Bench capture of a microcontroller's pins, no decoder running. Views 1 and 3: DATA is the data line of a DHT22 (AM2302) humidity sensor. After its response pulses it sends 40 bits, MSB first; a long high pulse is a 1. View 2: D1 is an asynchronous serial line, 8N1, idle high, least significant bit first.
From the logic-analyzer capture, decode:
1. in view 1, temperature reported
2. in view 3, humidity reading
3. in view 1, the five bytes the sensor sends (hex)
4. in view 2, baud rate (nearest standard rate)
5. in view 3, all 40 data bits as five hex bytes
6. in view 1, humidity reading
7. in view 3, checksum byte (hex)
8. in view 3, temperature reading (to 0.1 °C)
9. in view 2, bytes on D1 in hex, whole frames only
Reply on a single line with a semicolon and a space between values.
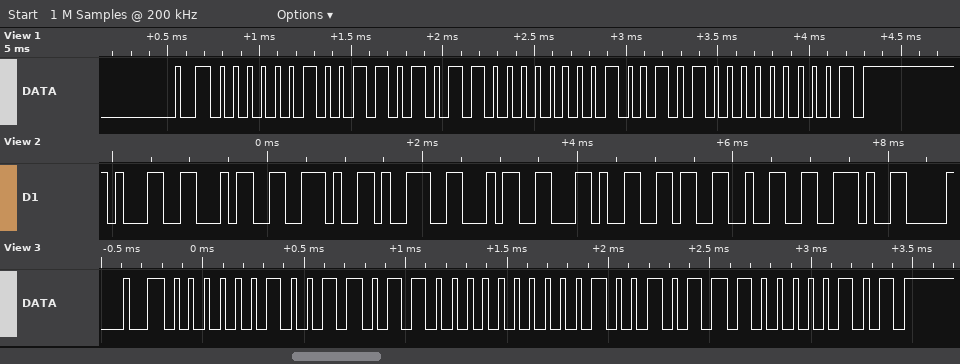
14.8 °C; 62.0 %; 02 6B 00 94 01; 9600 baud; 02 6C 00 97 05; 61.9 %; 0x05; 15.1 °C; 0x31 0x34 0x2E 0x39 0x34 0x2C 0x36 0x32 0x2E
